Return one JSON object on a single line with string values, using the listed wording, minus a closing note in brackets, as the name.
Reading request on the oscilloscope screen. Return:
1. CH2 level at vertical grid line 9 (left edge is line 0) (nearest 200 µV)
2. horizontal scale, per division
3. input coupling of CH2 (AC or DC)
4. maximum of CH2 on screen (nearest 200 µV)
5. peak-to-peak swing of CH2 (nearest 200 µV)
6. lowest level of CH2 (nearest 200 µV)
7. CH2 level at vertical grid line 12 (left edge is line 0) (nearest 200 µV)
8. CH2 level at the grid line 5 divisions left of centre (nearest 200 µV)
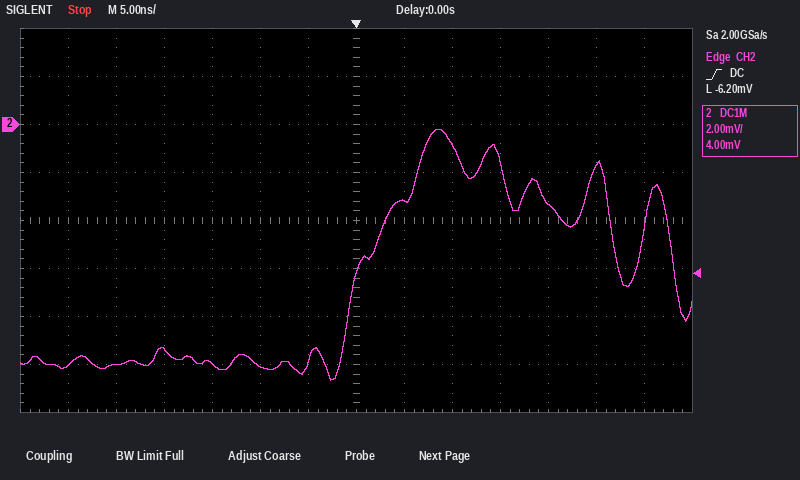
{"CH2 level at vertical grid line 9 (left edge is line 0)": "-800 µV", "horizontal scale, per division": "5 ns", "input coupling of CH2": "DC", "maximum of CH2 on screen": "-200 µV", "peak-to-peak swing of CH2": "10.4 mV", "lowest level of CH2": "-10.6 mV", "CH2 level at vertical grid line 12 (left edge is line 0)": "-1.8 mV", "CH2 level at the grid line 5 divisions left of centre": "-10.0 mV"}
